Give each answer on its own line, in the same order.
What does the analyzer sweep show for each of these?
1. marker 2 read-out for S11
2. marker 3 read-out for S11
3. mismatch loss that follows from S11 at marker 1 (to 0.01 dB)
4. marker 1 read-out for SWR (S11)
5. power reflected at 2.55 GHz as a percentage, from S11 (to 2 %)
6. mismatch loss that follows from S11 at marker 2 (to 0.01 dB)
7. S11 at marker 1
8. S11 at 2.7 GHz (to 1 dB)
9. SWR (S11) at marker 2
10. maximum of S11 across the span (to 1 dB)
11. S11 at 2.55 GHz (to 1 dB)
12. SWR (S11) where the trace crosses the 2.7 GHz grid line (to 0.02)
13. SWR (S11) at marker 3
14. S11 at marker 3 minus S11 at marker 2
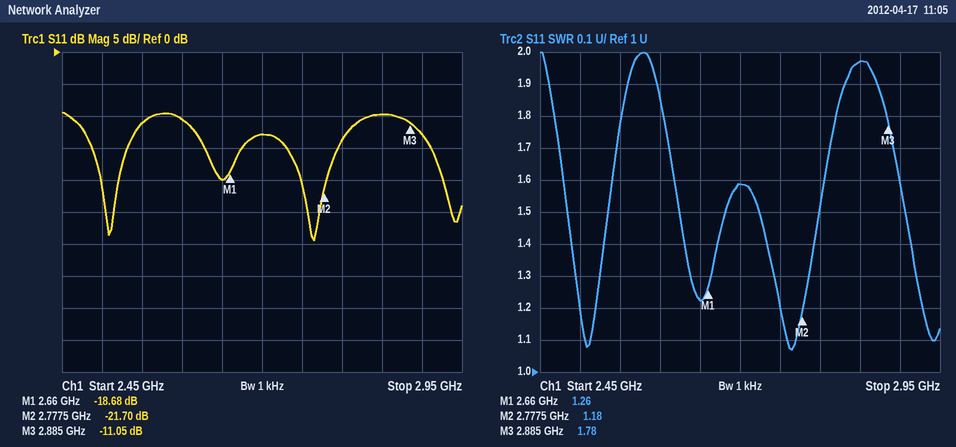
-21.70 dB
-11.05 dB
0.06 dB
1.26
8 %
0.03 dB
-18.68 dB
-13 dB
1.18
-9 dB
-11 dB
1.58
1.78
10.65 dB
